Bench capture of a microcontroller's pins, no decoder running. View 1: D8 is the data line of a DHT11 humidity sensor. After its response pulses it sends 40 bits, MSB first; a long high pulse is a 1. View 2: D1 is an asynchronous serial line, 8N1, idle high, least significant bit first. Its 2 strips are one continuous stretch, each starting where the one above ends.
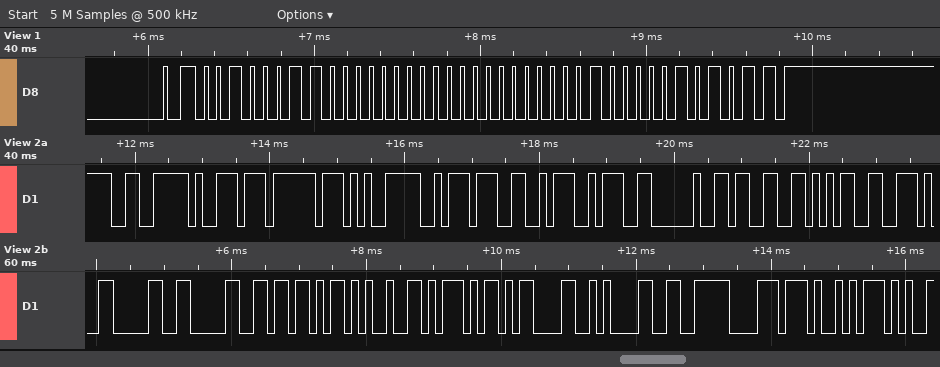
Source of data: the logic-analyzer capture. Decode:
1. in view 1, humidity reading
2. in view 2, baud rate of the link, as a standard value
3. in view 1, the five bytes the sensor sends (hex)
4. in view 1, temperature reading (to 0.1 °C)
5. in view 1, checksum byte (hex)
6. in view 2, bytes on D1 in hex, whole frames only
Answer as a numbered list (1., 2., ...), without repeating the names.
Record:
1. 35 %
2. 9600 baud
3. 23 00 00 08 2B
4. 0.8 °C
5. 0x2B
6. E6 B9 BF E5 BA A6 3A 20 33 35 2E 30 30 5B 25 5D 0D 0A E6 B8 A9
